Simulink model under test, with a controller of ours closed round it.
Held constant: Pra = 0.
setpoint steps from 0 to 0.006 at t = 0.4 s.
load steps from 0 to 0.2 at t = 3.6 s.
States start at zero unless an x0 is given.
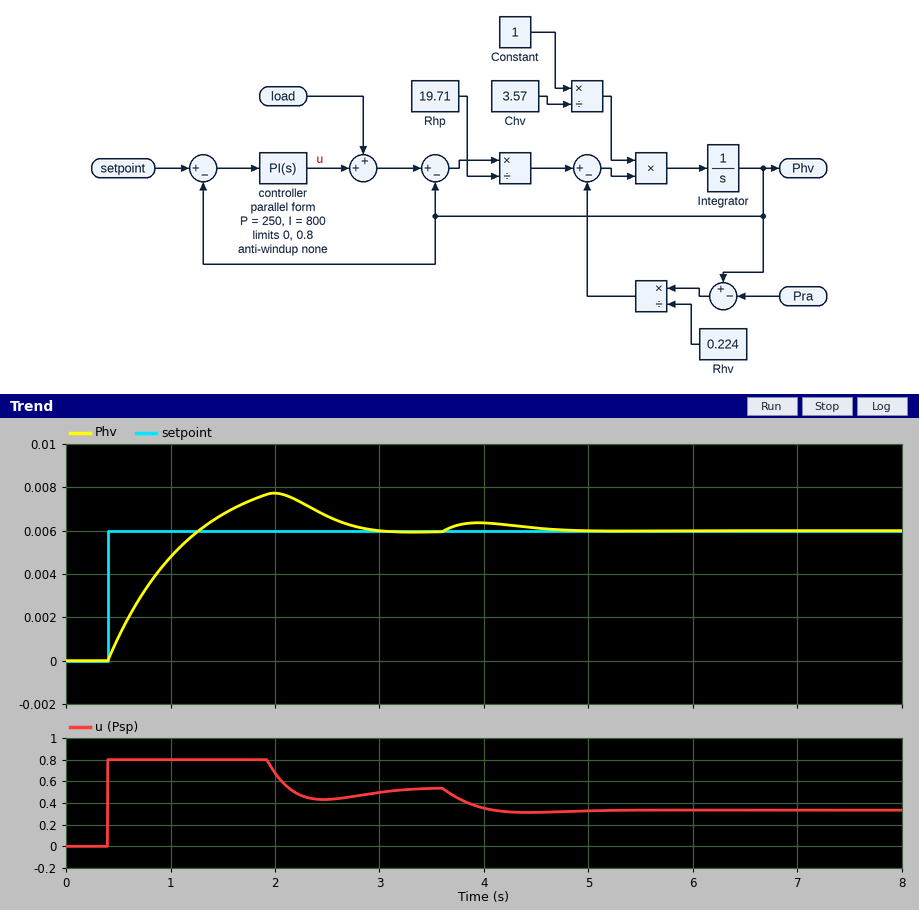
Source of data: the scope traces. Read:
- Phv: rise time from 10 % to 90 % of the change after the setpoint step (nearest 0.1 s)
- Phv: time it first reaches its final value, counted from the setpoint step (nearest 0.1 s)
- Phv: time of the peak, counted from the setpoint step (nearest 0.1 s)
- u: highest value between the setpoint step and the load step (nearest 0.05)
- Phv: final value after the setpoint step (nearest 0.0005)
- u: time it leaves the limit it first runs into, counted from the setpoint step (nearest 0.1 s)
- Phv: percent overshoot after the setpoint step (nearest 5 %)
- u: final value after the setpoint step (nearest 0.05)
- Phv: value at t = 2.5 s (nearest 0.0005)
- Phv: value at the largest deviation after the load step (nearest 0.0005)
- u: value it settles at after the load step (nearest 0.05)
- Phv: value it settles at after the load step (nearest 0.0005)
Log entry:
0.7 s
0.9 s
1.6 s
0.80
0.0060
1.5 s
30 %
0.55
0.0065
0.0065
0.35
0.0060
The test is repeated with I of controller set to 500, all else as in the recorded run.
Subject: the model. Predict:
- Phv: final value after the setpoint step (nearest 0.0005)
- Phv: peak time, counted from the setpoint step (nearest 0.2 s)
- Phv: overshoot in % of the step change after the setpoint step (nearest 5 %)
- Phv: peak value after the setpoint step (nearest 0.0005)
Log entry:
0.0060
1.4 s
20 %
0.0070
